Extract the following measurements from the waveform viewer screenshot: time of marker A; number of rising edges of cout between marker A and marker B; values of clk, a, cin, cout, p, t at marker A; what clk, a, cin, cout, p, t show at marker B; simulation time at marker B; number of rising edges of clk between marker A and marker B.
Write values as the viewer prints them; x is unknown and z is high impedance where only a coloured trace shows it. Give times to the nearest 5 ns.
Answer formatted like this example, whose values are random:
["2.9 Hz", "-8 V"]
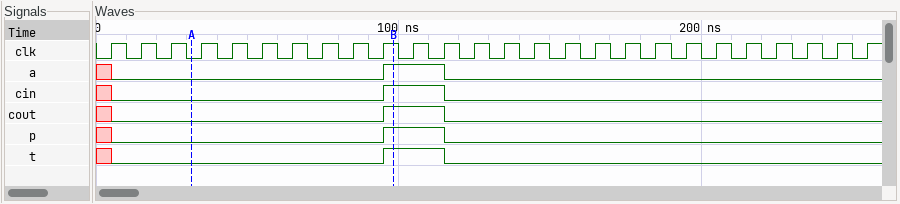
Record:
["30 ns", "1", "clk=0, a=0, cin=0, cout=0, p=0, t=0", "clk=1, a=1, cin=1, cout=1, p=1, t=1", "100 ns", "7"]
